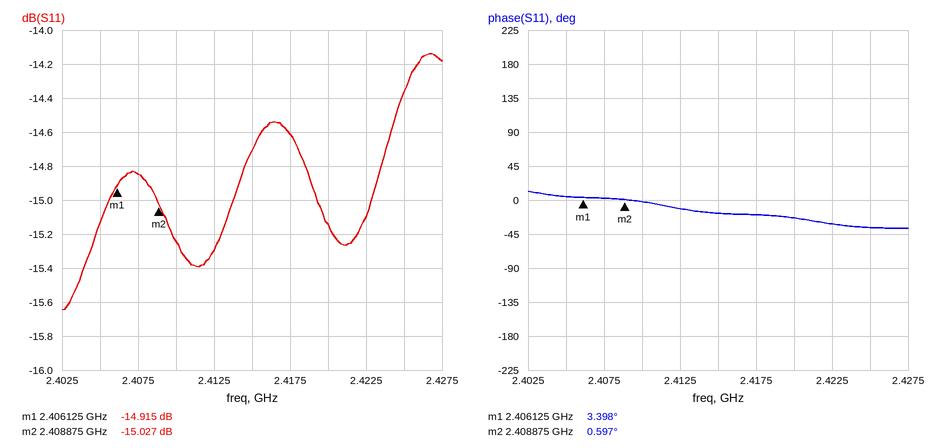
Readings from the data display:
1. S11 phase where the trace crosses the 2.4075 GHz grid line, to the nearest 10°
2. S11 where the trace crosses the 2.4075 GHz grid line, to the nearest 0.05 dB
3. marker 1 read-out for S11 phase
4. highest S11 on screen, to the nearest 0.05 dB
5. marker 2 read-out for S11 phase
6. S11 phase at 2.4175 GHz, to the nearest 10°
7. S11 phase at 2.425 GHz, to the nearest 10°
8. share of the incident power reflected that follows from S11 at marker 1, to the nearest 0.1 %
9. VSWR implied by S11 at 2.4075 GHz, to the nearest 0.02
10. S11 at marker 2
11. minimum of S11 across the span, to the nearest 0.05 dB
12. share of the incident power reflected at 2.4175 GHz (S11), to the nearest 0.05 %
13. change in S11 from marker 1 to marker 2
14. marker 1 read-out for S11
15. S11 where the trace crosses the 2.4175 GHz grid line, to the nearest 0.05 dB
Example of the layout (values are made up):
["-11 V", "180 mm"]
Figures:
["0°", "-14.85 dB", "3.398°", "-14.15 dB", "0.597°", "-20°", "-40°", "3.2 %", "1.44", "-15.027 dB", "-15.65 dB", "3.45 %", "-0.112 dB", "-14.915 dB", "-14.60 dB"]
